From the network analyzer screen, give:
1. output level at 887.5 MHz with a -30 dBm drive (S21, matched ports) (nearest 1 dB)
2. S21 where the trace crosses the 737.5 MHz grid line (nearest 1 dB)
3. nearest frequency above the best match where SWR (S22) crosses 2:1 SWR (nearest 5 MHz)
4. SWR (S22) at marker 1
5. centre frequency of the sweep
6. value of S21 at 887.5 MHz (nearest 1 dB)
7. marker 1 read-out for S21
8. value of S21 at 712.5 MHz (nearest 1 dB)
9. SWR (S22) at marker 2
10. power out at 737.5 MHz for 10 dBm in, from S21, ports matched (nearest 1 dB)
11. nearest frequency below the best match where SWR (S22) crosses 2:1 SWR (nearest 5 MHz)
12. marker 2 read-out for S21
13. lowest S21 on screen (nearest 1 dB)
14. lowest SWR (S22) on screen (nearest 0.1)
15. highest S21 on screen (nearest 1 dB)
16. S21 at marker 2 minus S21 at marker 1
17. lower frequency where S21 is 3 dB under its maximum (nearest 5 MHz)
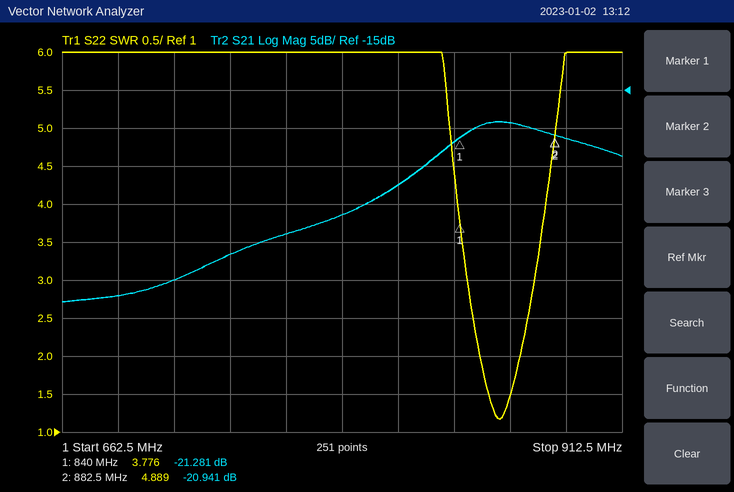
-51 dBm
-37 dB
865 MHz
3.776
787.5 MHz
-21 dB
-21.281 dB
-40 dB
4.889
-27 dBm
850 MHz
-20.941 dB
-43 dB
1.2
-19 dB
0.340 dB
835 MHz
